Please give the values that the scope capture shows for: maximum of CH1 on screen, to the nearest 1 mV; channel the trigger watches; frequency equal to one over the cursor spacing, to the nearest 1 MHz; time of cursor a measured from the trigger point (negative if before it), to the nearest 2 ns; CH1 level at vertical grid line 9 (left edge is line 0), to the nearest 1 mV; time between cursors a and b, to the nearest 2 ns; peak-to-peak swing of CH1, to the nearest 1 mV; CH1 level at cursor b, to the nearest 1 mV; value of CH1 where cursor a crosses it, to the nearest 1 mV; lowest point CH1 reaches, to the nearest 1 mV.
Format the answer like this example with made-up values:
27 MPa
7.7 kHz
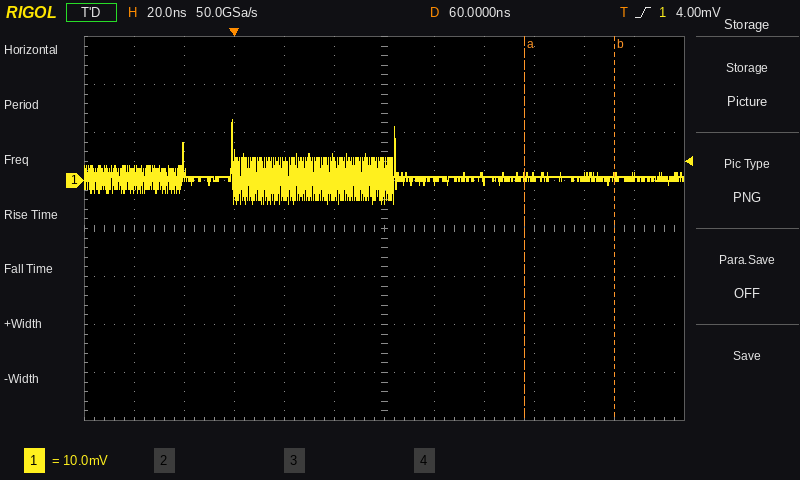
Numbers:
13 mV
CH1
28 MHz
+116 ns
1 mV
36 ns
18 mV
1 mV
1 mV
-5 mV
